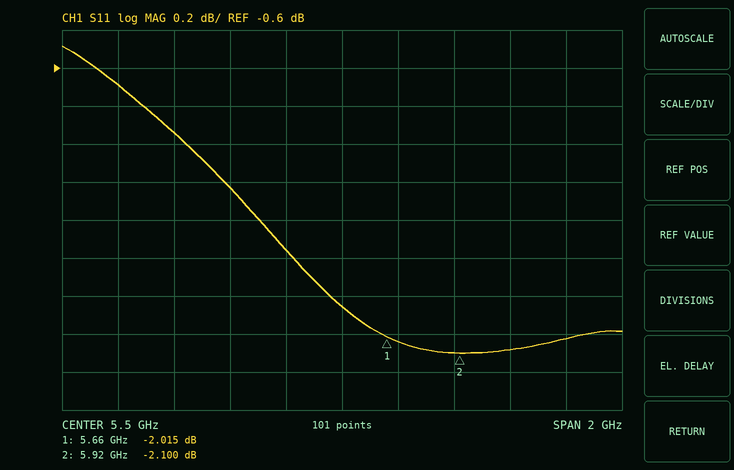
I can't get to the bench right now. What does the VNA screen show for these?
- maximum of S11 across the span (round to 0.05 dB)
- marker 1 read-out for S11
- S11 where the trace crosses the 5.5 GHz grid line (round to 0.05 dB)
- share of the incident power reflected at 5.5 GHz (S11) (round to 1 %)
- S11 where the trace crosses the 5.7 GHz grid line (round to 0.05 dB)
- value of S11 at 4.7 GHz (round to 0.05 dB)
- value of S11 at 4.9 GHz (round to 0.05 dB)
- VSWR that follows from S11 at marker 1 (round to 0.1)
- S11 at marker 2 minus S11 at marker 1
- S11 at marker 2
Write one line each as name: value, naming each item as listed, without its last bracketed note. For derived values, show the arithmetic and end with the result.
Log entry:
maximum of S11 across the span: -0.50 dB
marker 1 read-out for S11: -2.015 dB
S11 where the trace crosses the 5.5 GHz grid line: -1.85 dB
share of the incident power reflected at 5.5 GHz (S11): 10^(-1.85/10) ≈ 65 %
S11 where the trace crosses the 5.7 GHz grid line: -2.05 dB
value of S11 at 4.7 GHz: -0.70 dB
value of S11 at 4.9 GHz: -0.95 dB
VSWR that follows from S11 at marker 1: (1 + 0.7930)/(1 − 0.7930) ≈ 8.7
S11 at marker 2 minus S11 at marker 1: -2.1 − (-2.015) = -0.085 dB
S11 at marker 2: -2.100 dB
